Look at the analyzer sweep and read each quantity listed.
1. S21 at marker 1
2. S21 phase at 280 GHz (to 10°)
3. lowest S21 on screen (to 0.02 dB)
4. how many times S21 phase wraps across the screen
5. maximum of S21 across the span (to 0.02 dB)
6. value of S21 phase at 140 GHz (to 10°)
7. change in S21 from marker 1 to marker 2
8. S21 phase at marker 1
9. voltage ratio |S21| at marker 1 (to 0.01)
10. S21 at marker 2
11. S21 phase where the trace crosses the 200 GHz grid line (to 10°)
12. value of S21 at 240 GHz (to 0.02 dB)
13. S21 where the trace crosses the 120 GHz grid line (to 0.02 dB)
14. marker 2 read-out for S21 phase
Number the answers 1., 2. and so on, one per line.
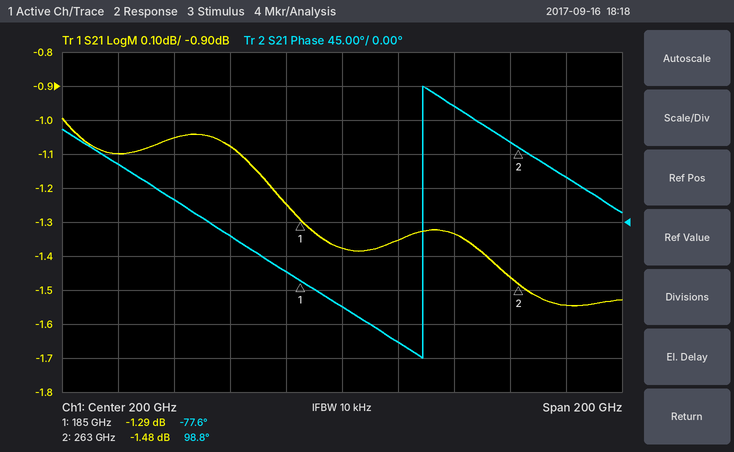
1. -1.29 dB
2. 60°
3. -1.54 dB
4. 1
5. -1.00 dB
6. 30°
7. -0.19 dB
8. -77.6°
9. 0.86
10. -1.48 dB
11. -110°
12. -1.34 dB
13. -1.10 dB
14. 98.8°
